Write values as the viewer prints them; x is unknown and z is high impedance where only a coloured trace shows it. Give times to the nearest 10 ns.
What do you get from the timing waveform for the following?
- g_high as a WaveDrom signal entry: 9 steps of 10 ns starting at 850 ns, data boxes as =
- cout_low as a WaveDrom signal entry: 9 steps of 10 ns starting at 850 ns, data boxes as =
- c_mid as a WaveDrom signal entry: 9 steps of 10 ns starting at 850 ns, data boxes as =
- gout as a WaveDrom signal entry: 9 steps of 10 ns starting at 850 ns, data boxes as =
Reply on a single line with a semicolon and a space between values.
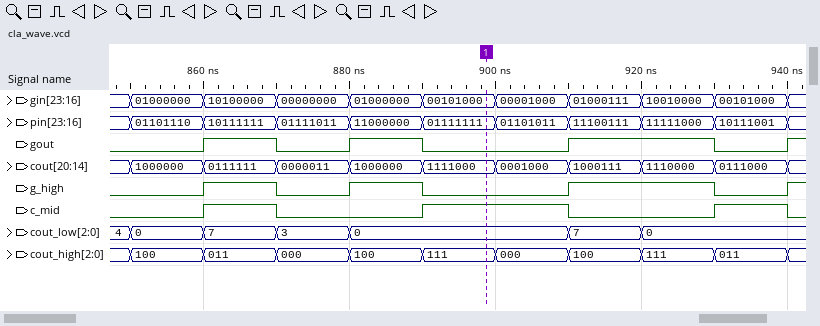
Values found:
{name: 'g_high', wave: '01010.1.0'}; {name: 'cout_low', wave: '====..==.', data: '0 7 3 0 7 0'}; {name: 'c_mid', wave: '010.1.0.1'}; {name: 'gout', wave: '01010.1.0'}
